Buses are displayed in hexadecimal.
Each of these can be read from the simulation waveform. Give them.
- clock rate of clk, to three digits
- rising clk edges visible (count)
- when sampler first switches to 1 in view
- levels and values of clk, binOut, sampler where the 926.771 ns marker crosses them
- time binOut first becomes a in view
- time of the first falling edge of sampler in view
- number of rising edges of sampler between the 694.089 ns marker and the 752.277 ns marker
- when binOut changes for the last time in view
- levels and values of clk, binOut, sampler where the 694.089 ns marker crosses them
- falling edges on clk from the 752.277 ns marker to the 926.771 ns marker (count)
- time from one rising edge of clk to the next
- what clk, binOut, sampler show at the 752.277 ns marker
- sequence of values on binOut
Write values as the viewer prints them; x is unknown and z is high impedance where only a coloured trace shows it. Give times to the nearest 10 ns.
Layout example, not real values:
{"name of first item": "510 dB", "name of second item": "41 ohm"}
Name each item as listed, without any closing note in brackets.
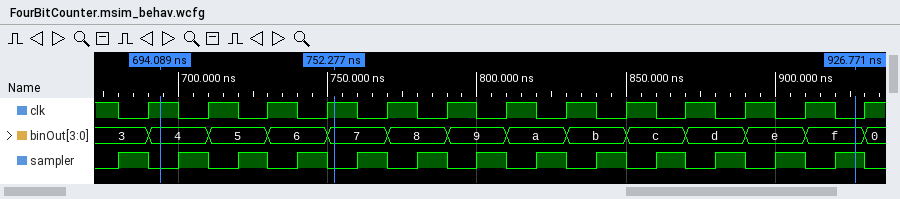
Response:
{"clock rate of clk, to three digits": "50.0 MHz", "rising clk edges visible": "13", "when sampler first switches to 1 in view": "680 ns", "levels and values of clk, binOut, sampler where the 926.771 ns marker crosses them": "clk=0, binOut=f, sampler=1", "time binOut first becomes a in view": "810 ns", "time of the first falling edge of sampler in view": "690 ns", "number of rising edges of sampler between the 694.089 ns marker and the 752.277 ns marker": "3", "when binOut changes for the last time in view": "930 ns", "levels and values of clk, binOut, sampler where the 694.089 ns marker crosses them": "clk=1, binOut=4, sampler=0", "falling edges on clk from the 752.277 ns marker to the 926.771 ns marker": "9", "time from one rising edge of clk to the next": "20 ns", "what clk, binOut, sampler show at the 752.277 ns marker": "clk=1, binOut=7, sampler=0", "sequence of values on binOut": "3, 4, 5, 6, 7, 8, 9, a, b, c, d, e, f, 0"}
